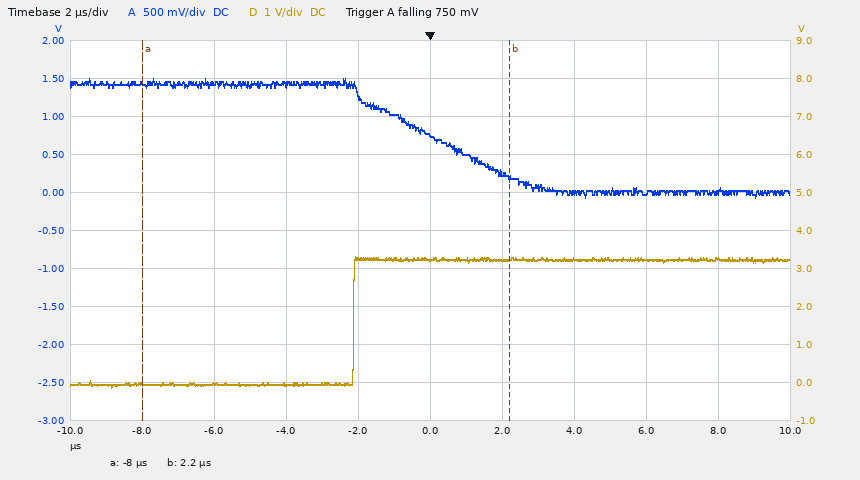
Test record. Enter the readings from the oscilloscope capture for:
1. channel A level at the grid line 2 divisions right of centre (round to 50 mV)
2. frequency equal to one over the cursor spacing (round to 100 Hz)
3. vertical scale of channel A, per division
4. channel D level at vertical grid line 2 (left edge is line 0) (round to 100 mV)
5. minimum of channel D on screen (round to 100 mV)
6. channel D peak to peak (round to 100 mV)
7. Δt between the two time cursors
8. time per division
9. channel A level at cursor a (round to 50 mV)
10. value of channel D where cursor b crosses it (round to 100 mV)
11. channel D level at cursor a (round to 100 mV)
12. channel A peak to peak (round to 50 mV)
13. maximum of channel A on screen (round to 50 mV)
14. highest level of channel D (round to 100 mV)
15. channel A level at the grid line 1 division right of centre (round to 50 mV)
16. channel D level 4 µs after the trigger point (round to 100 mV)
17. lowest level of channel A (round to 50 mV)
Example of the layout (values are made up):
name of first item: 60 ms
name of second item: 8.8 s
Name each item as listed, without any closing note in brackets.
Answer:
channel A level at the grid line 2 divisions right of centre: 0 mV
frequency equal to one over the cursor spacing: 98.0 kHz
vertical scale of channel A, per division: 500 mV
channel D level at vertical grid line 2 (left edge is line 0): 0.0 V
minimum of channel D on screen: -100 mV
channel D peak to peak: 3.4 V
Δt between the two time cursors: 10.2 µs
time per division: 2 µs
channel A level at cursor a: 1.45 V
value of channel D where cursor b crosses it: 3.2 V
channel D level at cursor a: 0.0 V
channel A peak to peak: 1.55 V
maximum of channel A on screen: 1.50 V
highest level of channel D: 3.3 V
channel A level at the grid line 1 division right of centre: 250 mV
channel D level 4 µs after the trigger point: 3.2 V
lowest level of channel A: -50 mV
